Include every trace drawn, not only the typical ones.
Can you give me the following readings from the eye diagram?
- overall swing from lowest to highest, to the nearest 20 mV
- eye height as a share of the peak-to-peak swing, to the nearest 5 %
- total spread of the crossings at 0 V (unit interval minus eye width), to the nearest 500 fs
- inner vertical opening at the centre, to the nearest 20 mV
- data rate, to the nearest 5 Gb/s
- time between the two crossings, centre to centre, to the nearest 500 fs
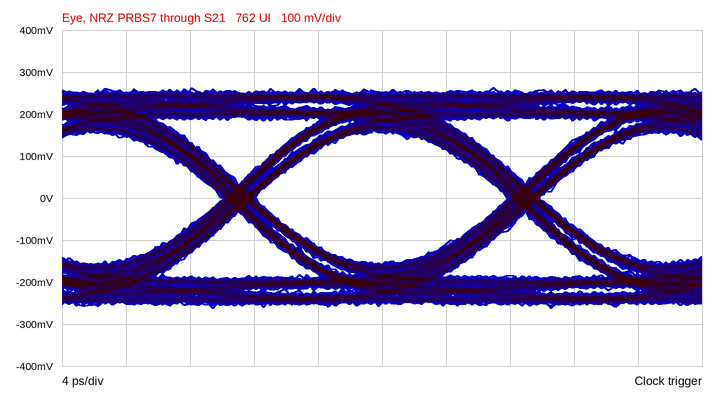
520 mV
60 %
2.0 ps
320 mV
55 Gb/s
18.0 ps
